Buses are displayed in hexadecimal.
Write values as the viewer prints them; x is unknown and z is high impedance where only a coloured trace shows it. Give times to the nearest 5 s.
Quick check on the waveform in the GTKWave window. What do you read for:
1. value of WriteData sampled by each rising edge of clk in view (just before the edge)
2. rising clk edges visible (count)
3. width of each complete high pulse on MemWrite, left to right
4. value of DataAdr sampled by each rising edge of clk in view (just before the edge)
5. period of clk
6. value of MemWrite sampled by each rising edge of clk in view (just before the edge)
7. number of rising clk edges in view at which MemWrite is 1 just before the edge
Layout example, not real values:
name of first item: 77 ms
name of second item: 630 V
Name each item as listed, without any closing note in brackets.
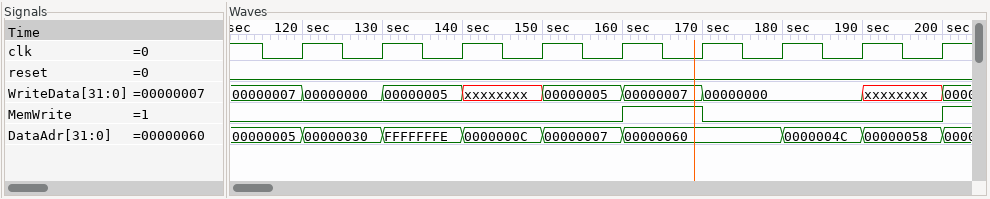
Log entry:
value of WriteData sampled by each rising edge of clk in view: 00000007, 00000000, 00000005, xxxxxxxx, 00000005, 00000007, 00000000, 00000000, xxxxxxxx
rising clk edges visible: 9
width of each complete high pulse on MemWrite, left to right: 10 s
value of DataAdr sampled by each rising edge of clk in view: 00000005, 00000030, FFFFFFFE, 0000000C, 00000007, 00000060, 00000060, 0000004C, 00000058
period of clk: 10 s
value of MemWrite sampled by each rising edge of clk in view: 0 0 0 0 0 1 0 0 0
number of rising clk edges in view at which MemWrite is 1 just before the edge: 1
